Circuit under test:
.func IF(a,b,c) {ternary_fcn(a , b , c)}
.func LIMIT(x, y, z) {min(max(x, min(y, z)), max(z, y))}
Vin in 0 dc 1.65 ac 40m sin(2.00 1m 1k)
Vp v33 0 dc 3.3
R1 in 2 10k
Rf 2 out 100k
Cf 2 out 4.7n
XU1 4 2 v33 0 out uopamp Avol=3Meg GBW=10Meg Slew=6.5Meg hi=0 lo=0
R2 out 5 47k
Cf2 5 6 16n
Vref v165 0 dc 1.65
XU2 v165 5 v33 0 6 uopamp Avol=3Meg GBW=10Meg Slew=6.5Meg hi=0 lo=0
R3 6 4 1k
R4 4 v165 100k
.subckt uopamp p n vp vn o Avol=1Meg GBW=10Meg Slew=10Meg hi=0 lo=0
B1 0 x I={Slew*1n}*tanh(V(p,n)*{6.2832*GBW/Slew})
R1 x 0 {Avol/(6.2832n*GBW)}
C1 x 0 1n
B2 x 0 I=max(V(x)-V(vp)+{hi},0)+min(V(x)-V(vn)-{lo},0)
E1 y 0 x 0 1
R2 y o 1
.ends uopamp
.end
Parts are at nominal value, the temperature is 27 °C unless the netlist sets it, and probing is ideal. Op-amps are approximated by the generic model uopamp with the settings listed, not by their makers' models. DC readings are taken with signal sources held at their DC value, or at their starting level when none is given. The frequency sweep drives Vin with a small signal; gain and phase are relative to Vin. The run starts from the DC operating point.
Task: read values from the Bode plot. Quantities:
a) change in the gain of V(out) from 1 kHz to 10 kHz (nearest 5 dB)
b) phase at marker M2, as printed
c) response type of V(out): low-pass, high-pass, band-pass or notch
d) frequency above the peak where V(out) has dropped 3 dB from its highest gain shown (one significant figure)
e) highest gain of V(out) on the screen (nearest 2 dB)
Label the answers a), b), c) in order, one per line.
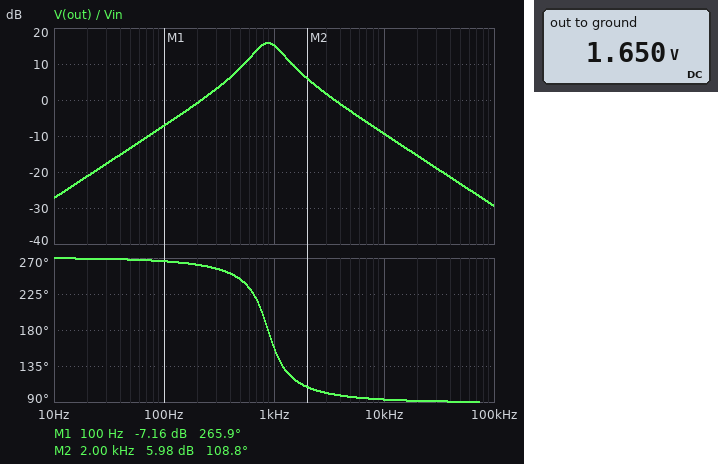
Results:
a) -25 dB
b) 108.8 deg
c) band-pass
d) 1 kHz
e) 16 dB
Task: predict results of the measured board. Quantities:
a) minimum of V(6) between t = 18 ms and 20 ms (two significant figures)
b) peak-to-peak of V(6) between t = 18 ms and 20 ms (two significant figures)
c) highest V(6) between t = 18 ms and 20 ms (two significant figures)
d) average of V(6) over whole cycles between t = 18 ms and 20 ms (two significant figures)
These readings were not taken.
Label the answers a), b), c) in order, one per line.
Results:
a) 2.0 V
b) 2.4 mV
c) 2.0 V
d) 2.0 V
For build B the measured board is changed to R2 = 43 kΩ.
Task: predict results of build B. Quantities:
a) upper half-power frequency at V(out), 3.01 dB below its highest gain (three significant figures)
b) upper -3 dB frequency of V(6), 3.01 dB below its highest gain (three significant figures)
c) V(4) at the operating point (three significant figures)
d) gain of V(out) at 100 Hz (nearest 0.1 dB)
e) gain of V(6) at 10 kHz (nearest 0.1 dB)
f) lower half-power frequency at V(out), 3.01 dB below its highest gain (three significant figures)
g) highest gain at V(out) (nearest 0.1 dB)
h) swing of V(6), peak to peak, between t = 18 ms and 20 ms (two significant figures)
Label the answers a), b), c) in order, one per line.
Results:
a) 1.25 kHz
b) 1.09 kHz
c) 1.65 V
d) -7.9 dB
e) -42.1 dB
f) 682 Hz
g) 15.5 dB
h) 2.7 mV
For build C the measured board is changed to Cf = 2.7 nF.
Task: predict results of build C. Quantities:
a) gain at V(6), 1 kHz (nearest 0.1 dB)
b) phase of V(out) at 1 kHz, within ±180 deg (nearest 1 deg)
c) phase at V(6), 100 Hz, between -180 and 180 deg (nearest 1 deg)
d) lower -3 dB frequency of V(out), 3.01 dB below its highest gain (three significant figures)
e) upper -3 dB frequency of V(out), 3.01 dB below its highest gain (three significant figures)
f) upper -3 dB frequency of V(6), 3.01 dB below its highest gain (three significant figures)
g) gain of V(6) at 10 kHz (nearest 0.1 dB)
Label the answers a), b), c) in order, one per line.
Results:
a) 3.1 dB
b) -156 deg
c) -3 deg
d) 833 Hz
e) 1.63 kHz
f) 1.38 kHz
g) -38.0 dB
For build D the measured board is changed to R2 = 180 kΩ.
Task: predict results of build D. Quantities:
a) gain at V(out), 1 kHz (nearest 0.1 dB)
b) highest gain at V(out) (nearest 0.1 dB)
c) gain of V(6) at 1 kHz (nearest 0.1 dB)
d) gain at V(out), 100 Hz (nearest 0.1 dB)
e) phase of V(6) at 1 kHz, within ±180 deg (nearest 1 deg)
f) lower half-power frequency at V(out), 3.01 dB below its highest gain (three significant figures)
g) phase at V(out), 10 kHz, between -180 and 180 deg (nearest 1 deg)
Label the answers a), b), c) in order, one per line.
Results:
a) 11.6 dB
b) 18.7 dB
c) -13.5 dB
d) 4.7 dB
e) -154 deg
f) 296 Hz
g) 92 deg
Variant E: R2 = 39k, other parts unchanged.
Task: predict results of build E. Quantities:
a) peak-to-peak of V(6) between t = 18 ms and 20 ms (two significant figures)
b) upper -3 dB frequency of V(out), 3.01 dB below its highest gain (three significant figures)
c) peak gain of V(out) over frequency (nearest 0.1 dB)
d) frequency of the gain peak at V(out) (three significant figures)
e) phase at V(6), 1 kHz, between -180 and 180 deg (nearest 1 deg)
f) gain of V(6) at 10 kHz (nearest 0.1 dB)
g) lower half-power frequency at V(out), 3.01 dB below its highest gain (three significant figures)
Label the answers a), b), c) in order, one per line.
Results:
a) 2.9 mV
b) 1.31 kHz
c) 15.2 dB
d) 970 Hz
e) -96 deg
f) -41.2 dB
g) 718 Hz
